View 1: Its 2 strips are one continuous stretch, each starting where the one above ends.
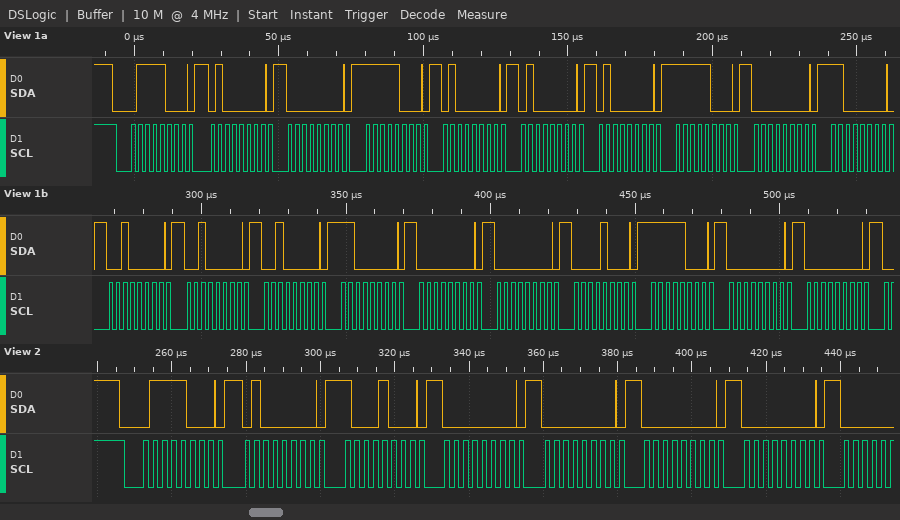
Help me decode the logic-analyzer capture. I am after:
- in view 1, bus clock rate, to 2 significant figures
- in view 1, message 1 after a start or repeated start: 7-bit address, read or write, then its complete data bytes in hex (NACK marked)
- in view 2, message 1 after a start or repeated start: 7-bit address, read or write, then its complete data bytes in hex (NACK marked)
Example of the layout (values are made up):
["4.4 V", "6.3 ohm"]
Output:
["400 kHz", "0x3C write: 40 00 F8 40 40 40 F8 00 C0 20 20 20 C0 00 00 08 F8 00 00", "0x3C write: 40 88 00 00 00 00"]
